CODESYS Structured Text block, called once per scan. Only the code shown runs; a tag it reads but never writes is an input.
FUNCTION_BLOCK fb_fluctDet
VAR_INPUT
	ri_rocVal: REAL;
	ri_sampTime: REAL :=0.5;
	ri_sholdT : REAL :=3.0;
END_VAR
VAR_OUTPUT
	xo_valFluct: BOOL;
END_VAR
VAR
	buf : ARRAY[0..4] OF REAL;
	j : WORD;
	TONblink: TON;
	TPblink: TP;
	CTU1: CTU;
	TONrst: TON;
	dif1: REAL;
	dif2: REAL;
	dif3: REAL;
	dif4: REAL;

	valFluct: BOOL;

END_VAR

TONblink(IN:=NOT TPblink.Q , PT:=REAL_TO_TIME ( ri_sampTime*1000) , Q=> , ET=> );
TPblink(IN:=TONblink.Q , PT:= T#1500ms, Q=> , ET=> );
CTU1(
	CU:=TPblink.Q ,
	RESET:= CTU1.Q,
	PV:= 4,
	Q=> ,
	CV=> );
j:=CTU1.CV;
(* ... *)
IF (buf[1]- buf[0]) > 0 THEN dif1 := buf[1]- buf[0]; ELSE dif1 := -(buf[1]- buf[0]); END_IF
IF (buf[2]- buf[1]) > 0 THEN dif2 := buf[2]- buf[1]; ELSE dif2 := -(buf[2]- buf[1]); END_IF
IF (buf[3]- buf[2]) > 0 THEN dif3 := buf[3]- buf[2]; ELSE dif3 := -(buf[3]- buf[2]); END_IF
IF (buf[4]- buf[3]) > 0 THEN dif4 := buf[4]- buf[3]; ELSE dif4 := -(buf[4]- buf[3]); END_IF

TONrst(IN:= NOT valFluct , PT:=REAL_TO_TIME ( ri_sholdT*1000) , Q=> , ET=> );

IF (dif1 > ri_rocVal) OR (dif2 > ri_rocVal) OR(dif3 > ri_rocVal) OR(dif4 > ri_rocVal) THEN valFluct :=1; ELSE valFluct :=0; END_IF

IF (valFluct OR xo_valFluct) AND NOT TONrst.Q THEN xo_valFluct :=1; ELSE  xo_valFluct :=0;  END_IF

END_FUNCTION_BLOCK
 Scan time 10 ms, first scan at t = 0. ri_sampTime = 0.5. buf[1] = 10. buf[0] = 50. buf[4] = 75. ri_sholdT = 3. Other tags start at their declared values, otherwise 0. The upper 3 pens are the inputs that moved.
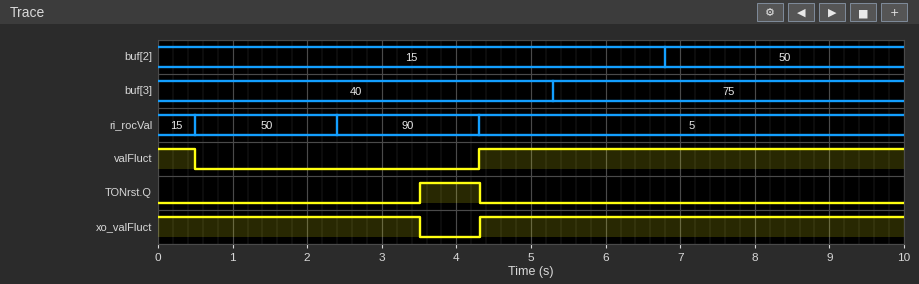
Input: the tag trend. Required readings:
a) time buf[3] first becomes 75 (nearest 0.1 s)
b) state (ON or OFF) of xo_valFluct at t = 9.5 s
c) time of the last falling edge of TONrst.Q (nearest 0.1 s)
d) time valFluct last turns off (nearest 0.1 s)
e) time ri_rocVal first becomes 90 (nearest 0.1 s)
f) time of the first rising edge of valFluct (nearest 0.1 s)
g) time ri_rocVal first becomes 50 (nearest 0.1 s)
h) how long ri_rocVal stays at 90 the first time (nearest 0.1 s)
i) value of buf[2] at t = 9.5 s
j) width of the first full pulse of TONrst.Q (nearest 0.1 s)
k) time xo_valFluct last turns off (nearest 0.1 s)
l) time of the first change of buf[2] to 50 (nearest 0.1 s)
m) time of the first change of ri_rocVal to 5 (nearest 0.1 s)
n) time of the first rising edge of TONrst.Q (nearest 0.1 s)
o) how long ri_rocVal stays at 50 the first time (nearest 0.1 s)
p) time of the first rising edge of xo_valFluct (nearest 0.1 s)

5.3 s
ON
4.3 s
0.5 s
2.4 s
4.3 s
0.5 s
1.9 s
50
0.8 s
3.5 s
6.8 s
4.3 s
3.5 s
1.9 s
4.3 s
